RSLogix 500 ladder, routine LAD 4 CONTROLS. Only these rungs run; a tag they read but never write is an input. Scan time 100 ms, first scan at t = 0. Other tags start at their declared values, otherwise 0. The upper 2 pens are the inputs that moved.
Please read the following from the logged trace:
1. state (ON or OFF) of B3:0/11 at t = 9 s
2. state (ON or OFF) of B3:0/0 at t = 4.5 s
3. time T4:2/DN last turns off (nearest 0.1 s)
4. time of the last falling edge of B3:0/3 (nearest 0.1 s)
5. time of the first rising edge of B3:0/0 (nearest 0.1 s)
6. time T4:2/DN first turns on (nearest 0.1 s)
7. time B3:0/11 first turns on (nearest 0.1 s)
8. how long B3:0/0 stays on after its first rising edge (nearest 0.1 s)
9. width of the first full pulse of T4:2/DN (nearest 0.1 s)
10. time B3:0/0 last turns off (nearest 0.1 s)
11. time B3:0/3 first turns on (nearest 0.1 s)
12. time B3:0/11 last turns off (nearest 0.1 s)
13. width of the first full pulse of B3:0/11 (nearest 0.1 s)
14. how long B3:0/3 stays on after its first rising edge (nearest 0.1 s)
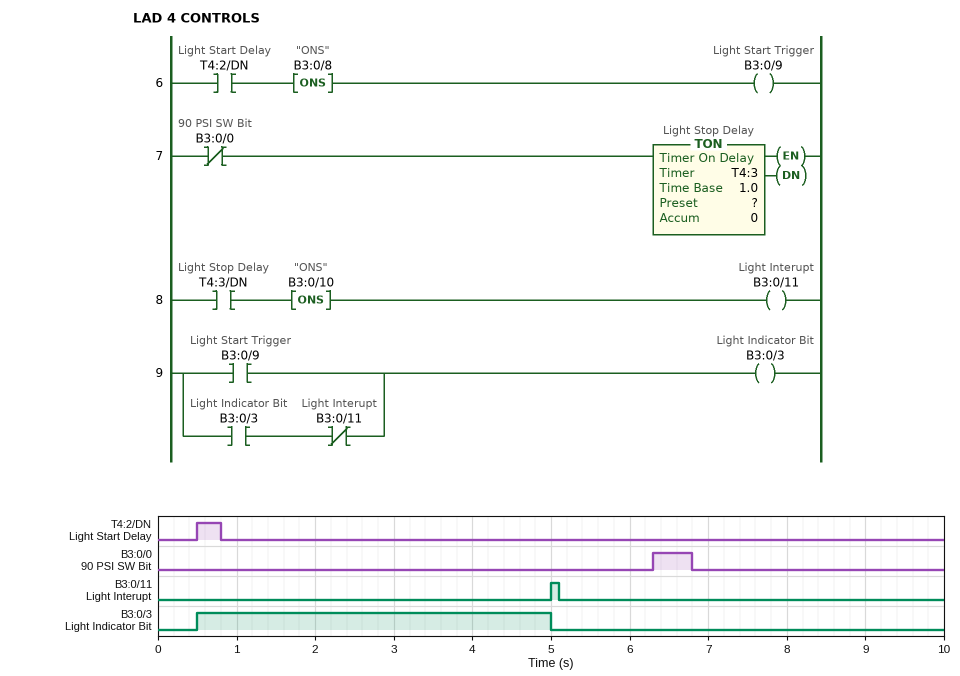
OFF
OFF
0.8 s
5.0 s
6.3 s
0.5 s
5.0 s
0.5 s
0.3 s
6.8 s
0.5 s
5.1 s
0.1 s
4.5 s
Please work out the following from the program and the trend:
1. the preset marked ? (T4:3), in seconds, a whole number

5 s
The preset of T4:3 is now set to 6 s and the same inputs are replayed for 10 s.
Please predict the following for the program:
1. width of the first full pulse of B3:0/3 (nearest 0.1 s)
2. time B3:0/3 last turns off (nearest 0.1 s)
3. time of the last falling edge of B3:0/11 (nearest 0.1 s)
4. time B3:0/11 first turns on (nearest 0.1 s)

5.5 s
6.0 s
6.1 s
6.0 s
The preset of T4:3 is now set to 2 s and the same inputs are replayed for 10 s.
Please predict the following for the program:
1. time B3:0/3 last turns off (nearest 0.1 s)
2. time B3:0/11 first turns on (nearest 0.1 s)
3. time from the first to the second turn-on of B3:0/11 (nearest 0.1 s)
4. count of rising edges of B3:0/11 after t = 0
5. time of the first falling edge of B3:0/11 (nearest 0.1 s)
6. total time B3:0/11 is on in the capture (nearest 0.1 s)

2.0 s
2.0 s
6.8 s
2
2.1 s
0.2 s
